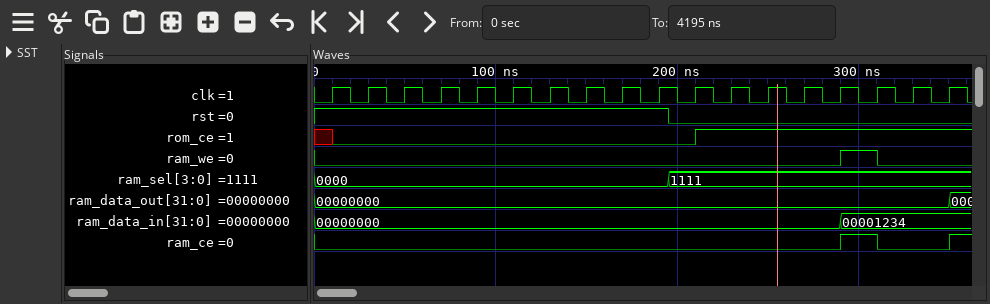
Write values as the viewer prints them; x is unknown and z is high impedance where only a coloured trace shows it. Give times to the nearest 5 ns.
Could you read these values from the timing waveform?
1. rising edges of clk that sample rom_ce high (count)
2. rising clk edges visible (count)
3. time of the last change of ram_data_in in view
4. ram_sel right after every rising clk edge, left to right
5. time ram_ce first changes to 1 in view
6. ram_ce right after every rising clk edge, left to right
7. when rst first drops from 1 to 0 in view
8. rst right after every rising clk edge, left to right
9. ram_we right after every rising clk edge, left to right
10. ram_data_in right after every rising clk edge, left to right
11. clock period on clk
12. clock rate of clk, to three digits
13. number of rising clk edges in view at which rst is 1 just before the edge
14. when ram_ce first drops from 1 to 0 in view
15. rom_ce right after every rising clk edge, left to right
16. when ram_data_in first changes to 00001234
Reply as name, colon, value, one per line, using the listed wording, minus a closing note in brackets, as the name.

rising edges of clk that sample rom_ce high: 7
rising clk edges visible: 18
time of the last change of ram_data_in in view: 290 ns
ram_sel right after every rising clk edge, left to right: 0000, 0000, 0000, 0000, 0000, 0000, 0000, 0000, 0000, 0000, 1111, 1111, 1111, 1111, 1111, 1111, 1111, 1111
time ram_ce first changes to 1 in view: 290 ns
ram_ce right after every rising clk edge, left to right: 0 0 0 0 0 0 0 0 0 0 0 0 0 0 1 0 0 1
when rst first drops from 1 to 0 in view: 195 ns
rst right after every rising clk edge, left to right: 1 1 1 1 1 1 1 1 1 1 0 0 0 0 0 0 0 0
ram_we right after every rising clk edge, left to right: 0 0 0 0 0 0 0 0 0 0 0 0 0 0 1 0 0 0
ram_data_in right after every rising clk edge, left to right: 00000000, 00000000, 00000000, 00000000, 00000000, 00000000, 00000000, 00000000, 00000000, 00000000, 00000000, 00000000, 00000000, 00000000, 00001234, 00001234, 00001234, 00001234
clock period on clk: 20 ns
clock rate of clk, to three digits: 50.0 MHz
number of rising clk edges in view at which rst is 1 just before the edge: 10
when ram_ce first drops from 1 to 0 in view: 310 ns
rom_ce right after every rising clk edge, left to right: 0 0 0 0 0 0 0 0 0 0 1 1 1 1 1 1 1 1
when ram_data_in first changes to 00001234: 290 ns
